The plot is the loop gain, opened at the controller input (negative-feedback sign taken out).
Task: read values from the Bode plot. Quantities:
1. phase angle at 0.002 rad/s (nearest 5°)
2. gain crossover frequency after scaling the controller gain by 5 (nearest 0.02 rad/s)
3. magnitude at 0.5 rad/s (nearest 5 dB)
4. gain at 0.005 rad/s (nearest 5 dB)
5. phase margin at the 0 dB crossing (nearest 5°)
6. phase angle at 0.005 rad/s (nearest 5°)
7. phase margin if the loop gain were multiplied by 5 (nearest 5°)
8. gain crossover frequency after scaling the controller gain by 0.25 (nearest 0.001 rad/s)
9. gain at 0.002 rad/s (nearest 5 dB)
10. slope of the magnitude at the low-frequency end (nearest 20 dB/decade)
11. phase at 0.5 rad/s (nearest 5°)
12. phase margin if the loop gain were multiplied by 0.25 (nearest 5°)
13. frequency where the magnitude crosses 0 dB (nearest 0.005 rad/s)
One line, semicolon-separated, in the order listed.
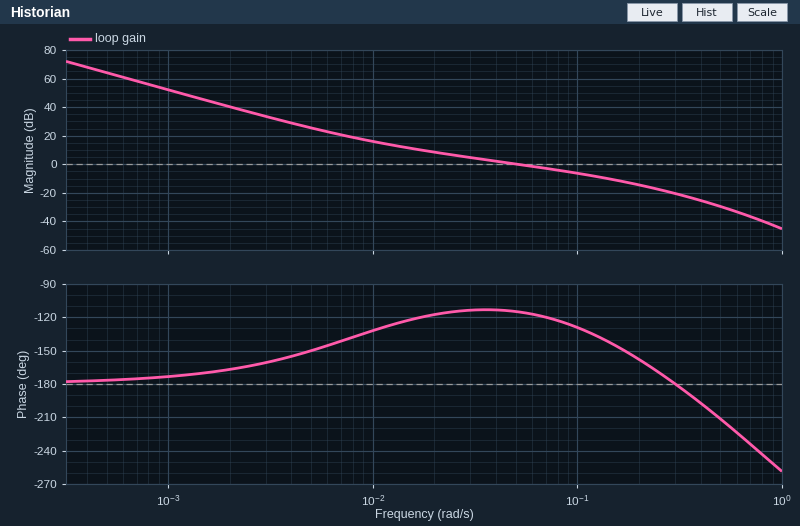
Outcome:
-165°; 0.20 rad/s; -30 dB; 25 dB; 65°; -150°; 25°; 0.014 rad/s; 40 dB; -40 dB/decade; -210°; 55°; 0.050 rad/s
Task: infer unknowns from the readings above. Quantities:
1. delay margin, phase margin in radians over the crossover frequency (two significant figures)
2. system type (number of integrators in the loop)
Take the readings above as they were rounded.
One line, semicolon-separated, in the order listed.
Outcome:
23 s; 2
